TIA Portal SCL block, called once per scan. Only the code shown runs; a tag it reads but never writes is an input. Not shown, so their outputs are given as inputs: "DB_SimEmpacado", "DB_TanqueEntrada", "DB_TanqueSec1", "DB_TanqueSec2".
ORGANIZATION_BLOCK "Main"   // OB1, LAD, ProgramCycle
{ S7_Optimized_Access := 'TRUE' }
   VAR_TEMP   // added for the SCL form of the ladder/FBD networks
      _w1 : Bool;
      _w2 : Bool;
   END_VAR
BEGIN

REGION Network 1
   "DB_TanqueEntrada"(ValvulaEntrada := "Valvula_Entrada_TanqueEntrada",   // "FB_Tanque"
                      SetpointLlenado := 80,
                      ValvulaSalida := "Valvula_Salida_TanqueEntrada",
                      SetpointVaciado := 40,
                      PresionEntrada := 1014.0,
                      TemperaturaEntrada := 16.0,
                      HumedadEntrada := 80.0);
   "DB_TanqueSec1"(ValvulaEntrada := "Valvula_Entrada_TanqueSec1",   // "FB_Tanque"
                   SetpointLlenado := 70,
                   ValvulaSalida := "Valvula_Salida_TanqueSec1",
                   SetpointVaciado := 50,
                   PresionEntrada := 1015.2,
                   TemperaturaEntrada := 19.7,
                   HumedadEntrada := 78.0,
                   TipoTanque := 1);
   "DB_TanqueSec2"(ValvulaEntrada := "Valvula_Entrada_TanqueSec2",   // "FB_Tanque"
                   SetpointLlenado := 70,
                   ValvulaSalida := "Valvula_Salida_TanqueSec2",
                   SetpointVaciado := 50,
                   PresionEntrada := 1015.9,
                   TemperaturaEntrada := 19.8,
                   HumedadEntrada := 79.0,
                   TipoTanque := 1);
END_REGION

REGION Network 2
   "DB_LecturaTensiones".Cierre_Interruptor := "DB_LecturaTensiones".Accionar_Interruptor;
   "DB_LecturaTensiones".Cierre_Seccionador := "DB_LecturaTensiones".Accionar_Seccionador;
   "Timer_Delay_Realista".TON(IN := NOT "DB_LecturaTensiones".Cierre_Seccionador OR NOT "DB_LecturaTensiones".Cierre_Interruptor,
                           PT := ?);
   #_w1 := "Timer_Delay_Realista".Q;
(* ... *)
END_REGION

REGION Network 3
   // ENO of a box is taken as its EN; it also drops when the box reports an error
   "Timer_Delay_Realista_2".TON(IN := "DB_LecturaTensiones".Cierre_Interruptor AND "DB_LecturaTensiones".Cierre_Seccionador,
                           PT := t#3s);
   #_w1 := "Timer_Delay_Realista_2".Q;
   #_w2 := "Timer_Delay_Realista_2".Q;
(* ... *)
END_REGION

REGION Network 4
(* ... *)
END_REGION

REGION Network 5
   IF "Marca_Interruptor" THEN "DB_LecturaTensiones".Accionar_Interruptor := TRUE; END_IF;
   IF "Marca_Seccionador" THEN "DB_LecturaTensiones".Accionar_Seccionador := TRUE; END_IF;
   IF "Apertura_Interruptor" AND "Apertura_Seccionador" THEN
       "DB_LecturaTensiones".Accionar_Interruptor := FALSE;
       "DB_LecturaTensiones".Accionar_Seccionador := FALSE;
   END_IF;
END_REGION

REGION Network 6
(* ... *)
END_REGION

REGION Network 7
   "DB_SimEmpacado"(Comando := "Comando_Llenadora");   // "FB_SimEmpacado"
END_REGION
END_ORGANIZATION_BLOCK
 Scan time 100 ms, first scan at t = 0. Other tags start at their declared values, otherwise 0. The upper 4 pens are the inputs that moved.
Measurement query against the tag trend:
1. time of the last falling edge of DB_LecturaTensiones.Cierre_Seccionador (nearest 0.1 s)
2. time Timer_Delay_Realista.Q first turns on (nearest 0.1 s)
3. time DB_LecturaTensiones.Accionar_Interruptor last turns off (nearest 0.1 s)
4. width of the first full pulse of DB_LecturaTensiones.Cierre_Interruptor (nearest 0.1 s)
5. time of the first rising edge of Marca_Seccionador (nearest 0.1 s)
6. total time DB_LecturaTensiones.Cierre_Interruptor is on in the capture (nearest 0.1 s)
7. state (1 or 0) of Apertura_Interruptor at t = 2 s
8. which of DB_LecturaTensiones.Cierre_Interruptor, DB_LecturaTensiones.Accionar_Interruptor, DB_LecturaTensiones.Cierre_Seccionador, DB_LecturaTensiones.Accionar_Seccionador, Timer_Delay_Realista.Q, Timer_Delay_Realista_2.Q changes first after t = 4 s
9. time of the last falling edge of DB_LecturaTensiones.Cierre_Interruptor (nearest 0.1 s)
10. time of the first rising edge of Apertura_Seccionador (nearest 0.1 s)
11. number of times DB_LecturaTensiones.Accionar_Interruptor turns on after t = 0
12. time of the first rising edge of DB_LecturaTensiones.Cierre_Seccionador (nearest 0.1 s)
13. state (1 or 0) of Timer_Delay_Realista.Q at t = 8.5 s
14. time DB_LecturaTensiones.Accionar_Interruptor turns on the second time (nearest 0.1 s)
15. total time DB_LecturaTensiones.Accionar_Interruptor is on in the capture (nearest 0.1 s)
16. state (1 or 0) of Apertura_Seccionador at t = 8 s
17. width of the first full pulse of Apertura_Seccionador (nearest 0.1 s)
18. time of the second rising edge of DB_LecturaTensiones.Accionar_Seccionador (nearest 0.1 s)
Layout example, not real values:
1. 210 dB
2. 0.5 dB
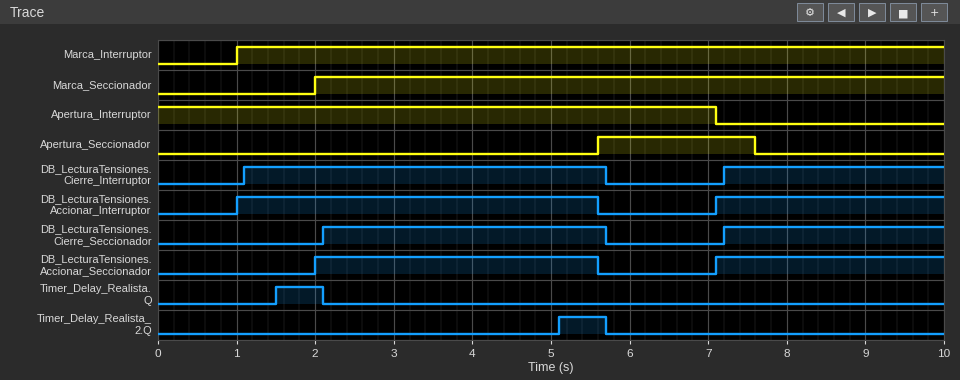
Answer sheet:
1. 5.7 s
2. 1.5 s
3. 5.6 s
4. 4.6 s
5. 2.0 s
6. 7.4 s
7. 1
8. Timer_Delay_Realista_2.Q
9. 5.7 s
10. 5.6 s
11. 2
12. 2.1 s
13. 0
14. 7.1 s
15. 7.5 s
16. 0
17. 2.0 s
18. 7.1 s
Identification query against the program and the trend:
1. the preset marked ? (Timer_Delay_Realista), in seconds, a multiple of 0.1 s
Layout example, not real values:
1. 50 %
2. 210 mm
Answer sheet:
1. 1.5 s
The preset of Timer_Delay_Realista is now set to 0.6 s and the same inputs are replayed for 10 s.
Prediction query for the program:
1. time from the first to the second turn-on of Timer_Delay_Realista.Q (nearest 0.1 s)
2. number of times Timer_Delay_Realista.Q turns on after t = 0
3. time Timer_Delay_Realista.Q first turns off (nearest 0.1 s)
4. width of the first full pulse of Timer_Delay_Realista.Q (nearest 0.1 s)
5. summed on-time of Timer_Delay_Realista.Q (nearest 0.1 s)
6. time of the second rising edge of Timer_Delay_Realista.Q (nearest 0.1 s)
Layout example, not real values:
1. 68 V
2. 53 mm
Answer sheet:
1. 5.7 s
2. 2
3. 2.1 s
4. 1.5 s
5. 2.4 s
6. 6.3 s
